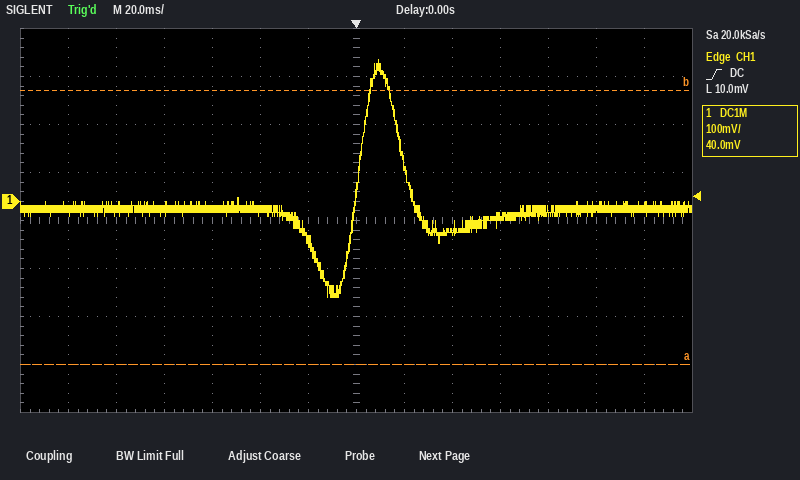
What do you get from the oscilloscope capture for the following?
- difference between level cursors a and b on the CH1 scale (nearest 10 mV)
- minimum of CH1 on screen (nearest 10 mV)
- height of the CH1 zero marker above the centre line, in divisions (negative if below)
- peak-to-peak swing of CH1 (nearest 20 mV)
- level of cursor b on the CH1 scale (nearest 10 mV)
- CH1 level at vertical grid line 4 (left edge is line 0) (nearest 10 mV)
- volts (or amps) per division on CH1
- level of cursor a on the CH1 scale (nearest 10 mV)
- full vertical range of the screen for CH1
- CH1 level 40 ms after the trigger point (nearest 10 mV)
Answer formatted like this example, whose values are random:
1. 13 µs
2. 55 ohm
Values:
1. 570 mV
2. -200 mV
3. +0.4 div
4. 500 mV
5. 230 mV
6. -20 mV
7. 100 mV
8. -340 mV
9. 800 mV
10. -60 mV
